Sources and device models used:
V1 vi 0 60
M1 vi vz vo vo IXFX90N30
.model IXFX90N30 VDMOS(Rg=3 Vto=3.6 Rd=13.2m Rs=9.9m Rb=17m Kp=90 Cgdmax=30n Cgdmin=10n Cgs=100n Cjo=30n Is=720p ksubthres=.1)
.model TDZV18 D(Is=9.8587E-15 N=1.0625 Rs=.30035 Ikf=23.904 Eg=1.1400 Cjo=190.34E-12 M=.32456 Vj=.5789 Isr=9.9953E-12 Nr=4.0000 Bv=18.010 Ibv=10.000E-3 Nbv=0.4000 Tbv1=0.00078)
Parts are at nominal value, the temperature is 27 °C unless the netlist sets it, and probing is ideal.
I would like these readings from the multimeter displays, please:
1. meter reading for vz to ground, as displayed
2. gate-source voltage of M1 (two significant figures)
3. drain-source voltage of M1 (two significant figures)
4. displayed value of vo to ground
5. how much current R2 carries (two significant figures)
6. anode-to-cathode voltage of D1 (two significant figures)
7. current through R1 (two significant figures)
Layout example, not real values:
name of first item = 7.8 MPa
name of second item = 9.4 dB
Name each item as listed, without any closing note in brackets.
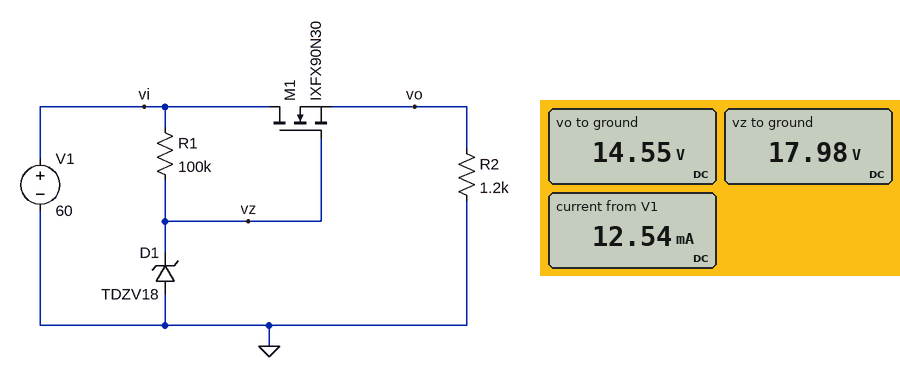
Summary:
meter reading for vz to ground, as displayed = 17.98 V
gate-source voltage of M1 = 3.4 V
drain-source voltage of M1 = 45 V
displayed value of vo to ground = 14.55 V
how much current R2 carries = 12 mA
anode-to-cathode voltage of D1 = -18 V
current through R1 = 420 µA
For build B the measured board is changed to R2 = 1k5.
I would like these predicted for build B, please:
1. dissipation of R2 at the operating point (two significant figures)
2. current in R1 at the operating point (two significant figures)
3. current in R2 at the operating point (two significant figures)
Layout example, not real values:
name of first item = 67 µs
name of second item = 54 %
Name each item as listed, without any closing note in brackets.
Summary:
dissipation of R2 at the operating point = 140 mW
current in R1 at the operating point = 420 µA
current in R2 at the operating point = 9.7 mA
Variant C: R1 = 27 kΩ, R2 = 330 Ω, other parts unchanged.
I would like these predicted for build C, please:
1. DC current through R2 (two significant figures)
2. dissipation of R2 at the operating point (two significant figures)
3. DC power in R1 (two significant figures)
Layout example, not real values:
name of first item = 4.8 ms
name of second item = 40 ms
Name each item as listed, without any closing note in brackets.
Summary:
DC current through R2 = 44 mA
dissipation of R2 at the operating point = 640 mW
DC power in R1 = 65 mW
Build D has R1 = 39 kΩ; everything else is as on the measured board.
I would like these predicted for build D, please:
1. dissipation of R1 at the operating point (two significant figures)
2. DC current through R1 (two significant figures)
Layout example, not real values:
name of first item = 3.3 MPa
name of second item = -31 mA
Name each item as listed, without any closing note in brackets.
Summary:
dissipation of R1 at the operating point = 45 mW
DC current through R1 = 1.1 mA
